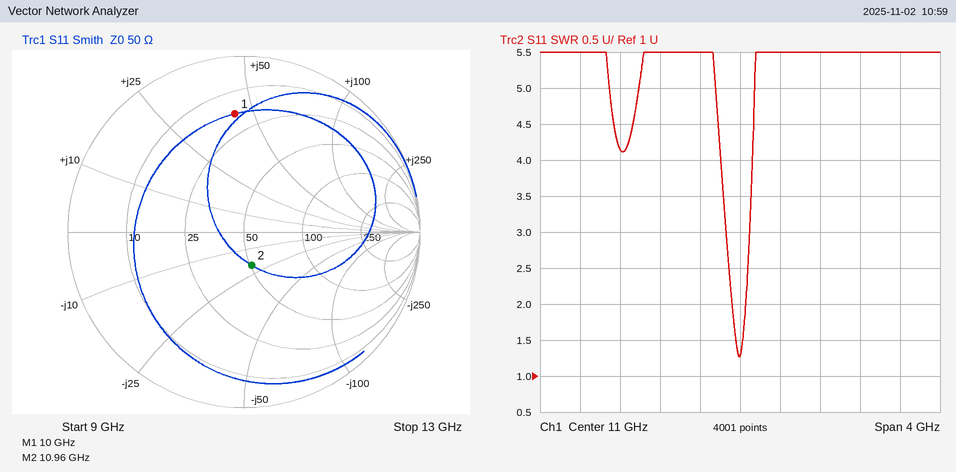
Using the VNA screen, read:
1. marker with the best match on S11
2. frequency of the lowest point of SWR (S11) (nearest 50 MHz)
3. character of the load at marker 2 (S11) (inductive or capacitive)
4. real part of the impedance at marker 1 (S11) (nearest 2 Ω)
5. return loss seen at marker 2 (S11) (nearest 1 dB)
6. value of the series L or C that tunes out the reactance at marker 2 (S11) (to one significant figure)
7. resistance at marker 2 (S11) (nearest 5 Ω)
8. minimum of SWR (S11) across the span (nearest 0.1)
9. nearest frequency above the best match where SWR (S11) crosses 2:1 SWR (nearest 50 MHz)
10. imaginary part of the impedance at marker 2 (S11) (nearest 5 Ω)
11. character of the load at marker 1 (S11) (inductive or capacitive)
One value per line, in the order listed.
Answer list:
marker 2
11.00 GHz
capacitive
18 Ω
14 dB
300 pH
50 Ω
1.3
11.05 GHz
-20 Ω
inductive
